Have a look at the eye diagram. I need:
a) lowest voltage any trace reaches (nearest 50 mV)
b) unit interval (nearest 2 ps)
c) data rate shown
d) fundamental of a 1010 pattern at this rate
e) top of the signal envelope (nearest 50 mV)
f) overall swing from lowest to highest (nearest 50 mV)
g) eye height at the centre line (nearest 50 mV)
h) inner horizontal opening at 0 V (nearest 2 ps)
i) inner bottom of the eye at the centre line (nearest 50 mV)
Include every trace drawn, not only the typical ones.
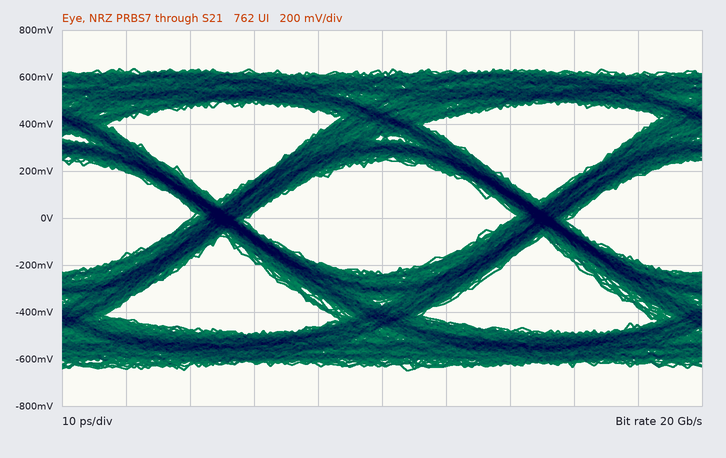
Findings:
-650 mV
50 ps
20 Gb/s
10 GHz
650 mV
1.30 V
500 mV
42 ps
-250 mV
